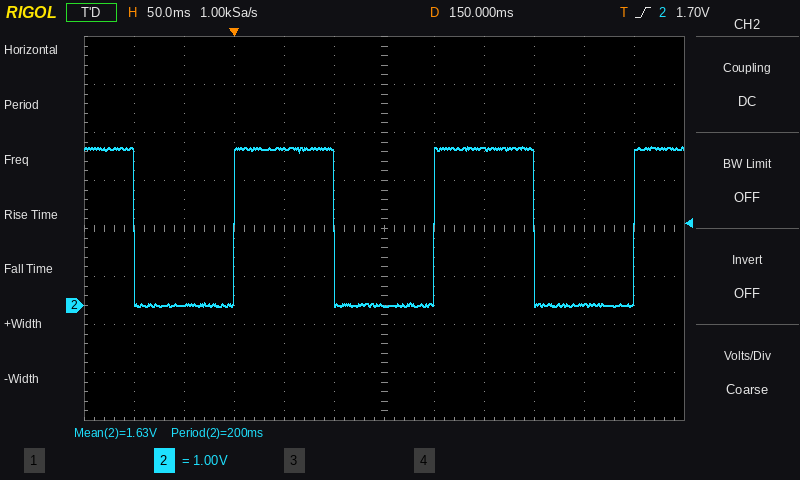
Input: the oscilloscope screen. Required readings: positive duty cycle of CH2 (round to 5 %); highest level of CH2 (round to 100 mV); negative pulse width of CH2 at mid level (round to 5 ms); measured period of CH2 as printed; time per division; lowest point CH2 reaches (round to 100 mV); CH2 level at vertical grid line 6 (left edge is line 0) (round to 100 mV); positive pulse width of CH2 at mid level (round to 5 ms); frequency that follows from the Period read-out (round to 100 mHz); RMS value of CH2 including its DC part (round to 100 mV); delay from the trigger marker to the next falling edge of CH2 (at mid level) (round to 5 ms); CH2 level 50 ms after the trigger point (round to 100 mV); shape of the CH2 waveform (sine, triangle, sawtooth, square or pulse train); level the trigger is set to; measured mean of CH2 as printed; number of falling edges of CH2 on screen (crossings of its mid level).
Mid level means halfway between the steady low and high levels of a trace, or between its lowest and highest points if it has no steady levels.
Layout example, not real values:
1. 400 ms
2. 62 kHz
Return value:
1. 50 %
2. 3.3 V
3. 100 ms
4. 200 ms
5. 50 ms
6. 0.0 V
7. 0.0 V
8. 100 ms
9. 5.0 Hz
10. 2.3 V
11. 100 ms
12. 3.3 V
13. square
14. 1.70 V
15. 1.63 V
16. 3
